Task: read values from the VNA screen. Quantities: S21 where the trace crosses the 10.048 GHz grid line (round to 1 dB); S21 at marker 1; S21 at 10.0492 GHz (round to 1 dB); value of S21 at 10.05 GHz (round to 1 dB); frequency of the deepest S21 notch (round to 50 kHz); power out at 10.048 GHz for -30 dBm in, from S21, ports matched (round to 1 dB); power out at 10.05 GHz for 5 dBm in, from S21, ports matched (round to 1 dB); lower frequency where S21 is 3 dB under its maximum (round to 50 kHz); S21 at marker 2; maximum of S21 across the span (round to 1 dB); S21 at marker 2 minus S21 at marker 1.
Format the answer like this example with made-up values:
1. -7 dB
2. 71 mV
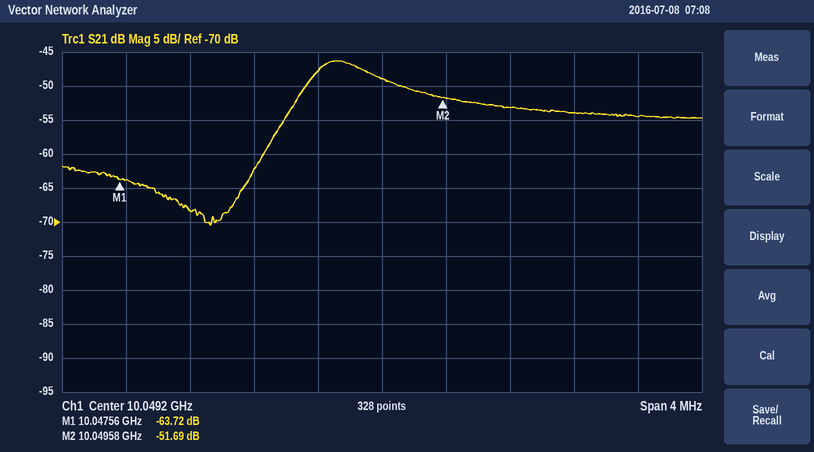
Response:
1. -68 dB
2. -63.72 dB
3. -49 dB
4. -53 dB
5. 10.04815 GHz
6. -98 dBm
7. -48 dBm
8. 10.04875 GHz
9. -51.69 dB
10. -46 dB
11. 12.03 dB
